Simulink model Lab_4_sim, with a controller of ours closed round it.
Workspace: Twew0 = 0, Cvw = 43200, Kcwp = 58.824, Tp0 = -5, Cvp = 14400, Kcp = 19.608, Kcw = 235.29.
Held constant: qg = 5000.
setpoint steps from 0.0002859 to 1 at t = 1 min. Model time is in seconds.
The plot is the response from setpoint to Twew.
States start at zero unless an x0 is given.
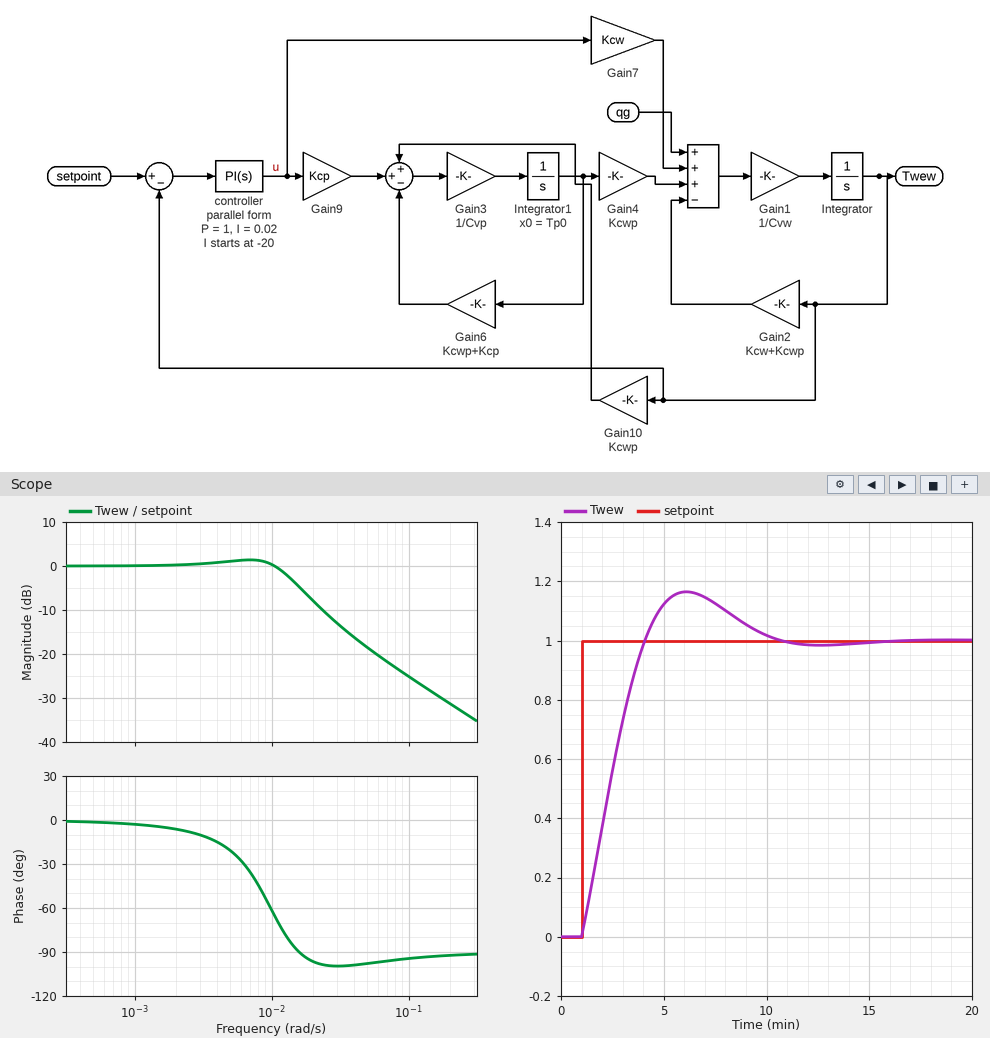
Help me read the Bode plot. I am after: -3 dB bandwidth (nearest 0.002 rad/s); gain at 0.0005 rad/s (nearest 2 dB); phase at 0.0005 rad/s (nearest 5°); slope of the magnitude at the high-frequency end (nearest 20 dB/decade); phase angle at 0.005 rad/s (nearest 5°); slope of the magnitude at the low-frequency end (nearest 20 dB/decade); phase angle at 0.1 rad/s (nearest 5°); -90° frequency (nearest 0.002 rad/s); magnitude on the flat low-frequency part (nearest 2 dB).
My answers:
0.014 rad/s
0 dB
0°
-20 dB/decade
-20°
0 dB/decade
-95°
0.016 rad/s
0 dB
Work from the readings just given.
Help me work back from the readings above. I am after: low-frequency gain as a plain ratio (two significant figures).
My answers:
1.0
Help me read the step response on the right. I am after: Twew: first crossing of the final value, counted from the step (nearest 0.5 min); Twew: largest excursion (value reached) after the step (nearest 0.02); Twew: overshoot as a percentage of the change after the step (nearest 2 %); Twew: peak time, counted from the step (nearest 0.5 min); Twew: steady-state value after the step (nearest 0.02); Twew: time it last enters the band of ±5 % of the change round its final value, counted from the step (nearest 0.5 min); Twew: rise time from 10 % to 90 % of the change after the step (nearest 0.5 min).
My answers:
3.0 min
1.16
16 %
5.0 min
1.00
8.0 min
2.5 min
